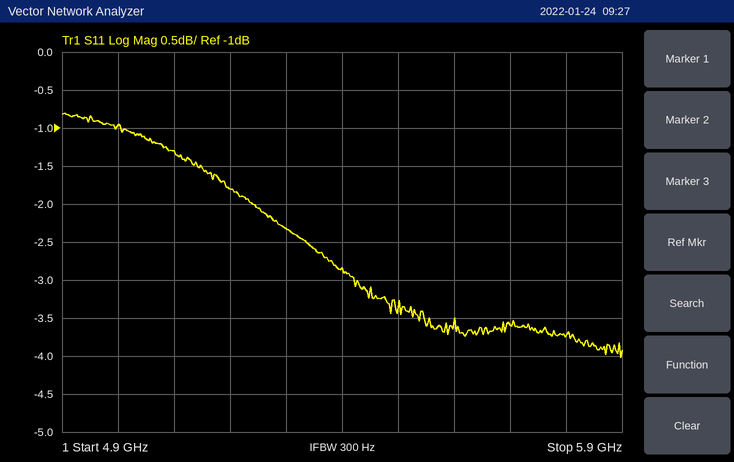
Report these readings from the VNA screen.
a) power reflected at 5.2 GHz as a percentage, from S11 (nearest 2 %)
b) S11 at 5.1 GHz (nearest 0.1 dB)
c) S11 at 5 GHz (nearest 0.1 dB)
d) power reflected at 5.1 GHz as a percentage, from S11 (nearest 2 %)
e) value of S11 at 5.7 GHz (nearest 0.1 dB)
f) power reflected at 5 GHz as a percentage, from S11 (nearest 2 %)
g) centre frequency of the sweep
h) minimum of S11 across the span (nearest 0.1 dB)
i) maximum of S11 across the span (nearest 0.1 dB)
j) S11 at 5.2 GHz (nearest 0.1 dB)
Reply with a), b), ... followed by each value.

a) 66 %
b) -1.3 dB
c) -1.0 dB
d) 74 %
e) -3.6 dB
f) 80 %
g) 5.4 GHz
h) -4.0 dB
i) -0.8 dB
j) -1.8 dB
